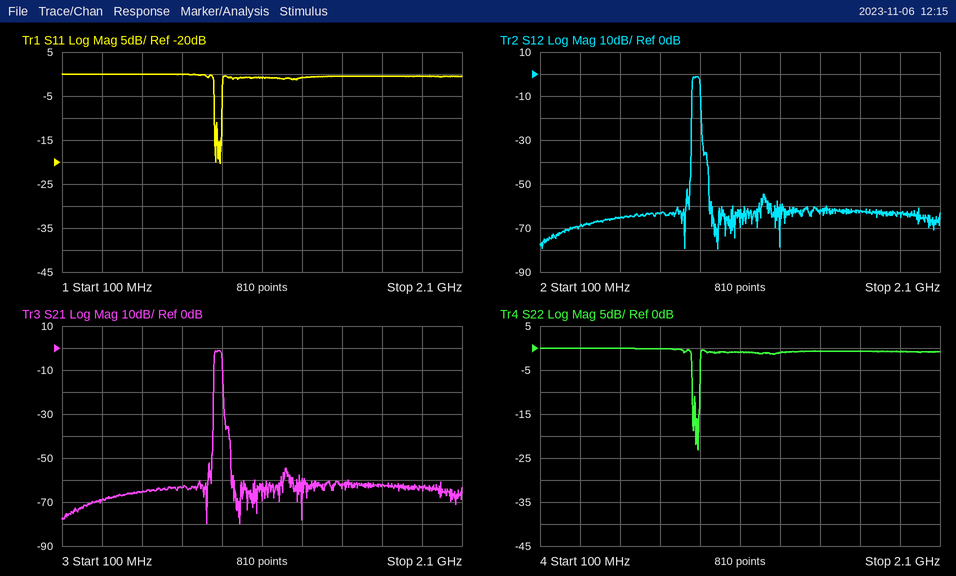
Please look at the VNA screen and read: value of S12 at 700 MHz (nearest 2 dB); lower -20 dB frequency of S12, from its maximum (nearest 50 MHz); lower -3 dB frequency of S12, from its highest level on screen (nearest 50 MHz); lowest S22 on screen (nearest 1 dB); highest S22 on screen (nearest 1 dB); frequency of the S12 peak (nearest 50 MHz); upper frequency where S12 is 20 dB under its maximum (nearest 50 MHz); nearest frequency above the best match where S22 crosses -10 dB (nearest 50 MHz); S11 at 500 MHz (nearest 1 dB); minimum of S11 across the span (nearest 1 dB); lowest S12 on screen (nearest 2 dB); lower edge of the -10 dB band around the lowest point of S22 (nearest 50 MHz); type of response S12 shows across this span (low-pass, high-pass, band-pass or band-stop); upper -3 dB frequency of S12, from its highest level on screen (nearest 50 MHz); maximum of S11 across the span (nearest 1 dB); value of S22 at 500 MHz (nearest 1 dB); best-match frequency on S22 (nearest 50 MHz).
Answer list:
-64 dB
850 MHz
850 MHz
-23 dB
0 dB
900 MHz
900 MHz
900 MHz
0 dB
-20 dB
-80 dB
850 MHz
band-pass
900 MHz
0 dB
0 dB
900 MHz
